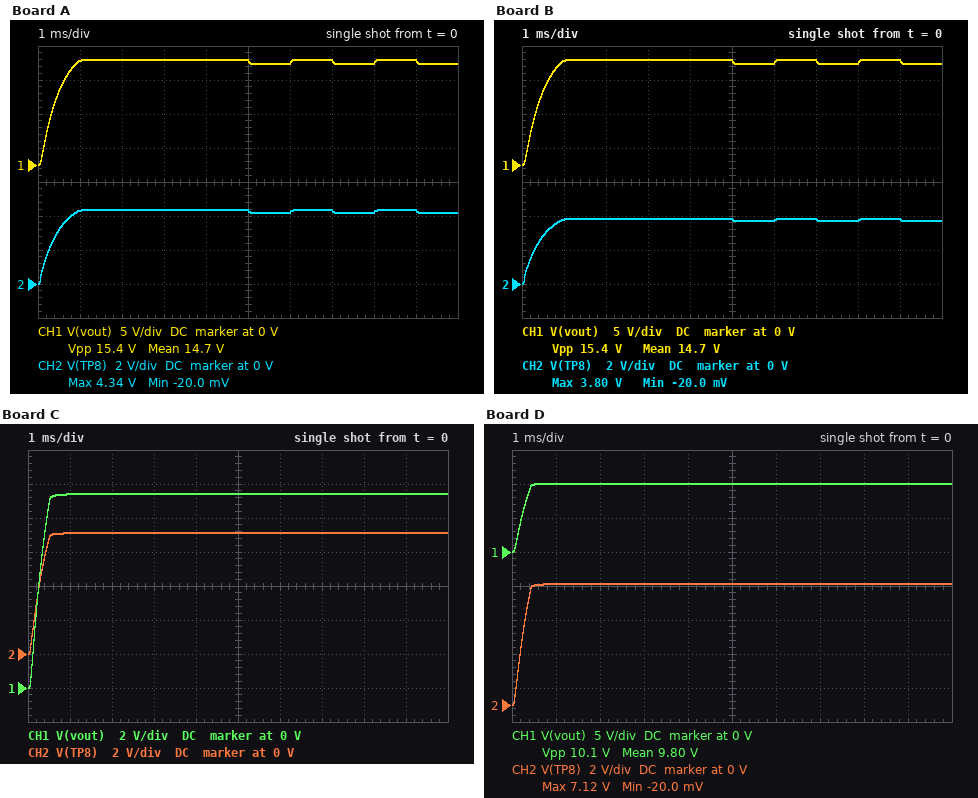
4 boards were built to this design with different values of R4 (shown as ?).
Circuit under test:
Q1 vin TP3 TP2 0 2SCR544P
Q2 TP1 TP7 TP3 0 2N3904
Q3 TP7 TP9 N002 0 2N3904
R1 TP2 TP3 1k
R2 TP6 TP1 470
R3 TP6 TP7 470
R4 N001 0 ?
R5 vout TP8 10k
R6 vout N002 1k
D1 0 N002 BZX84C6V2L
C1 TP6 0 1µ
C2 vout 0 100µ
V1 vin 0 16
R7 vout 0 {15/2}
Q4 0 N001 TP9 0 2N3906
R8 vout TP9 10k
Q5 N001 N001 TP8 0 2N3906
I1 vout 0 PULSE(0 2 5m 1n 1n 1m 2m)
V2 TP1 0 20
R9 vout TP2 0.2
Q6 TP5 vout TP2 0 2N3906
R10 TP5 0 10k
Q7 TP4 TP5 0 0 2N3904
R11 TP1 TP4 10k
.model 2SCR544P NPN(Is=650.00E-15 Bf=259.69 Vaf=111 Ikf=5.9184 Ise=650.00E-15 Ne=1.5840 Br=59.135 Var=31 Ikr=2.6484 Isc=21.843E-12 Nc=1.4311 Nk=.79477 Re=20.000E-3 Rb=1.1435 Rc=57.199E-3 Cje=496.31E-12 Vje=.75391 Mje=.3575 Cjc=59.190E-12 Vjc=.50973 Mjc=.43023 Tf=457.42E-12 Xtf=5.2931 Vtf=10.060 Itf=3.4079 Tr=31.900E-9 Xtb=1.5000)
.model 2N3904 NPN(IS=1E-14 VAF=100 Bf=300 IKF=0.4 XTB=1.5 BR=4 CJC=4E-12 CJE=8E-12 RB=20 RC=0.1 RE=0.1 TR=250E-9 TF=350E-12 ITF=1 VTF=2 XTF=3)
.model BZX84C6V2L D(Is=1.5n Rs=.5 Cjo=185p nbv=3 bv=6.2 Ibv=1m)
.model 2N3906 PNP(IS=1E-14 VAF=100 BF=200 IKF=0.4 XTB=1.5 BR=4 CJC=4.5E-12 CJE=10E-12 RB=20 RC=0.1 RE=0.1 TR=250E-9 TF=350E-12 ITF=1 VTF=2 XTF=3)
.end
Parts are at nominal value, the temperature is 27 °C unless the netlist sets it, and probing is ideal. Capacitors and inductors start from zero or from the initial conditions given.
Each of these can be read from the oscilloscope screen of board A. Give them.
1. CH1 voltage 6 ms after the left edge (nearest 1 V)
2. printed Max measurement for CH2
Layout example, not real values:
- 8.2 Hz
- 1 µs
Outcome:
- 15 V
- 4.34 V
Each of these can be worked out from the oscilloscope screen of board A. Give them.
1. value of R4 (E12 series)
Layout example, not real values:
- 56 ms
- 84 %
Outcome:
- 3.3 kΩ
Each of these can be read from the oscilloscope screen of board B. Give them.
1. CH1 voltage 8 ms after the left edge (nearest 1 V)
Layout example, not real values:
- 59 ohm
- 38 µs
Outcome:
- 15 V
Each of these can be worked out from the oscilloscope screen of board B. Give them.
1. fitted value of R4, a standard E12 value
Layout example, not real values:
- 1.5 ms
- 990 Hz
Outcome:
- 2.7 kΩ
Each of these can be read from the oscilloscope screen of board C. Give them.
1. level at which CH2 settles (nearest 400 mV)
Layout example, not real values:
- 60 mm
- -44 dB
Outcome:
- 7.2 V
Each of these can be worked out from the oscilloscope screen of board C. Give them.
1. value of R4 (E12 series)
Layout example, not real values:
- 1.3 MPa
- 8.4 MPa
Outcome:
- 15 kΩ
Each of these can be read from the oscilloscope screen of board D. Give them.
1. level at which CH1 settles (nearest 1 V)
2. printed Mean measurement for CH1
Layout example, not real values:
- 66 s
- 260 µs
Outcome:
- 10 V
- 9.80 V
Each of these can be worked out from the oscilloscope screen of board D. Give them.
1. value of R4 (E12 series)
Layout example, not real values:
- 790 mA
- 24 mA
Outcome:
- 22 kΩ
